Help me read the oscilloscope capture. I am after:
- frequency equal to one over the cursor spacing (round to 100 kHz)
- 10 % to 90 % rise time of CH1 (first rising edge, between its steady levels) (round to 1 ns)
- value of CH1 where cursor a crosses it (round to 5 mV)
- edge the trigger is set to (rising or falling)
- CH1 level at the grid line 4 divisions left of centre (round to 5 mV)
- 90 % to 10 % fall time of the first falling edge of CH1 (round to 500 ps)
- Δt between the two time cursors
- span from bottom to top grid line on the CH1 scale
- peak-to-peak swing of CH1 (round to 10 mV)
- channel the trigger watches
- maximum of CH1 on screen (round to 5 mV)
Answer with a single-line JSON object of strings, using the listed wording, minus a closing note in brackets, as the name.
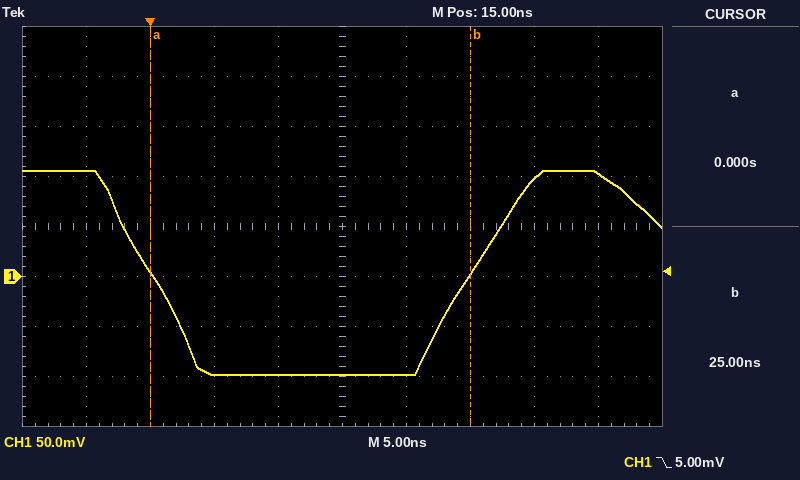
{"frequency equal to one over the cursor spacing": "40.0 MHz", "10 % to 90 % rise time of CH1 (first rising edge, between its steady levels)": "8 ns", "value of CH1 where cursor a crosses it": "5 mV", "edge the trigger is set to": "falling", "CH1 level at the grid line 4 divisions left of centre": "105 mV", "90 % to 10 % fall time of the first falling edge of CH1": "6.5 ns", "Δt between the two time cursors": "25.0 ns", "span from bottom to top grid line on the CH1 scale": "400 mV", "peak-to-peak swing of CH1": "200 mV", "channel the trigger watches": "CH1", "maximum of CH1 on screen": "105 mV"}
